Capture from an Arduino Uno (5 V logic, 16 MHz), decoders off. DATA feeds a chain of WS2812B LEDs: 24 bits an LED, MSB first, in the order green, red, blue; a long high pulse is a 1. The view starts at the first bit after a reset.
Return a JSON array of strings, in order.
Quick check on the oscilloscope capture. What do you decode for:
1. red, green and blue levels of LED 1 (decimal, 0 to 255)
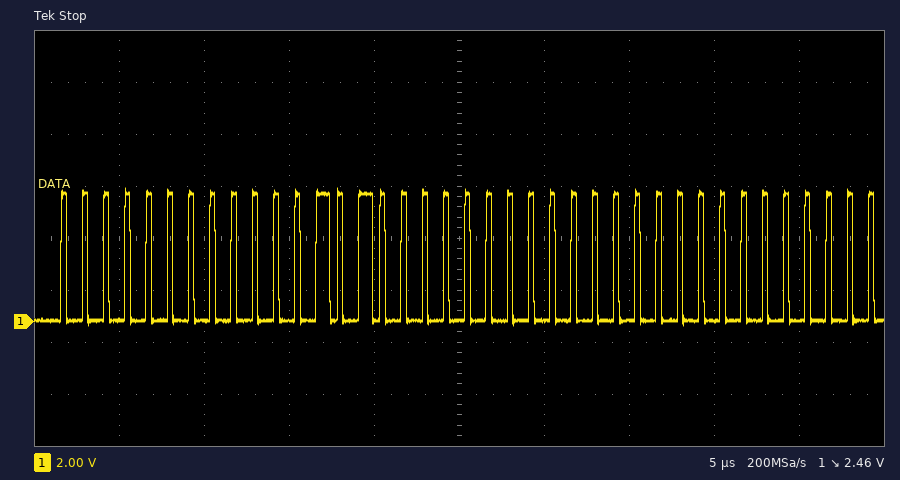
["10, 0, 0"]
